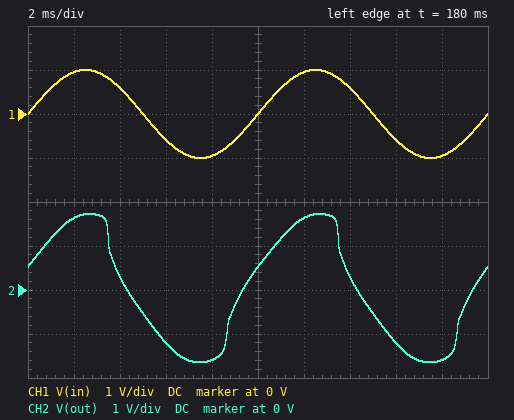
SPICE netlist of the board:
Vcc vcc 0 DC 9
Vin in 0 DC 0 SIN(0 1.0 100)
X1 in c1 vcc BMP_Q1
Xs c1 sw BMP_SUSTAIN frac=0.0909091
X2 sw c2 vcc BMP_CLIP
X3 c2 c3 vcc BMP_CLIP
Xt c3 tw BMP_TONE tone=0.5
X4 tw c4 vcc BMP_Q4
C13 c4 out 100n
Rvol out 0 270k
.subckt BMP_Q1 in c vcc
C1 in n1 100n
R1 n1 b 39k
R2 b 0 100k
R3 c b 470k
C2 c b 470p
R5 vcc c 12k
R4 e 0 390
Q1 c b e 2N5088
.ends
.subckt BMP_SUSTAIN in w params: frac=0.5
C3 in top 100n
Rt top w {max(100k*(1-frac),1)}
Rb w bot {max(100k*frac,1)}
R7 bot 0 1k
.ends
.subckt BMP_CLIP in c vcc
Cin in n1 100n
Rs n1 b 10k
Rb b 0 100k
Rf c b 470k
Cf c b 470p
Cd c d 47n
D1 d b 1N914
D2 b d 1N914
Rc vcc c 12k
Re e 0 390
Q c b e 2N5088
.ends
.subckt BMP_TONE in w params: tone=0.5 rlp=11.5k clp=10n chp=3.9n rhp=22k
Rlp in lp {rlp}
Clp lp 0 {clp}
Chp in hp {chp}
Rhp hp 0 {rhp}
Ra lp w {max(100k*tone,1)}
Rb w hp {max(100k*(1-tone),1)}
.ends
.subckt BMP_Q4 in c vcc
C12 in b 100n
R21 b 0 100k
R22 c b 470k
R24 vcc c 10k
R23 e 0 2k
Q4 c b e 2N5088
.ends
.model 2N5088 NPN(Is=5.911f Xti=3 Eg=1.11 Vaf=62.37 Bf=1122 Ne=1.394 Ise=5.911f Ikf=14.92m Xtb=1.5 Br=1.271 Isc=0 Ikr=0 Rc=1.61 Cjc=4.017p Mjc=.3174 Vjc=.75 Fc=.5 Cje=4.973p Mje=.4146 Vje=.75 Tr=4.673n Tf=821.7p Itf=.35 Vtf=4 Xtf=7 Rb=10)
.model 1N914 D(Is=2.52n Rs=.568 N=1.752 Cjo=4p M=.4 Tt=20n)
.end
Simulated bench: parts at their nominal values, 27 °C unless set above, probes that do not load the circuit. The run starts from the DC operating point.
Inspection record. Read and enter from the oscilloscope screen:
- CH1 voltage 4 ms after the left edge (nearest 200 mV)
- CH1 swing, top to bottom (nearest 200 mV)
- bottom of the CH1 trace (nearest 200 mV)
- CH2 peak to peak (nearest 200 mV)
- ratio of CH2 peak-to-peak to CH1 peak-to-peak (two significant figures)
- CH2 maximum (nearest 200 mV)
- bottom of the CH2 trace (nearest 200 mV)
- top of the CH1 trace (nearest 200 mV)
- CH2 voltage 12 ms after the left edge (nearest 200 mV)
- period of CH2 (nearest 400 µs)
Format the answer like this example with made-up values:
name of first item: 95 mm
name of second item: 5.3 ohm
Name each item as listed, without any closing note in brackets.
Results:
CH1 voltage 4 ms after the left edge: 600 mV
CH1 swing, top to bottom: 2.0 V
bottom of the CH1 trace: -1.0 V
CH2 peak to peak: 3.4 V
ratio of CH2 peak-to-peak to CH1 peak-to-peak: 1.7
CH2 maximum: 1.8 V
bottom of the CH2 trace: -1.6 V
top of the CH1 trace: 1.0 V
CH2 voltage 12 ms after the left edge: 1.6 V
period of CH2: 10.0 ms
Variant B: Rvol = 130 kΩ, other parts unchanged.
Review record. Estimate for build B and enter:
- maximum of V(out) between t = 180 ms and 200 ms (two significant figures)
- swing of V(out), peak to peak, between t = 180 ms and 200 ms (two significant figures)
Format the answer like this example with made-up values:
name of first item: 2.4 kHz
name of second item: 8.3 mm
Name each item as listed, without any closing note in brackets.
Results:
maximum of V(out) between t = 180 ms and 200 ms: 1.6 V
swing of V(out), peak to peak, between t = 180 ms and 200 ms: 3.2 V
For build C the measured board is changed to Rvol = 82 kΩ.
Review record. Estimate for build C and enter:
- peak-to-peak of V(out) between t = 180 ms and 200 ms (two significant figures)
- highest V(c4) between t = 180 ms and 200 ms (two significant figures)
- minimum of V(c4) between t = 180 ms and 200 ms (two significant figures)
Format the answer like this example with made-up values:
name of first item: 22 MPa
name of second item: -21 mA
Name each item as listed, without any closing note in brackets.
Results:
peak-to-peak of V(out) between t = 180 ms and 200 ms: 3.0 V
highest V(c4) between t = 180 ms and 200 ms: 8.2 V
minimum of V(c4) between t = 180 ms and 200 ms: 4.9 V
